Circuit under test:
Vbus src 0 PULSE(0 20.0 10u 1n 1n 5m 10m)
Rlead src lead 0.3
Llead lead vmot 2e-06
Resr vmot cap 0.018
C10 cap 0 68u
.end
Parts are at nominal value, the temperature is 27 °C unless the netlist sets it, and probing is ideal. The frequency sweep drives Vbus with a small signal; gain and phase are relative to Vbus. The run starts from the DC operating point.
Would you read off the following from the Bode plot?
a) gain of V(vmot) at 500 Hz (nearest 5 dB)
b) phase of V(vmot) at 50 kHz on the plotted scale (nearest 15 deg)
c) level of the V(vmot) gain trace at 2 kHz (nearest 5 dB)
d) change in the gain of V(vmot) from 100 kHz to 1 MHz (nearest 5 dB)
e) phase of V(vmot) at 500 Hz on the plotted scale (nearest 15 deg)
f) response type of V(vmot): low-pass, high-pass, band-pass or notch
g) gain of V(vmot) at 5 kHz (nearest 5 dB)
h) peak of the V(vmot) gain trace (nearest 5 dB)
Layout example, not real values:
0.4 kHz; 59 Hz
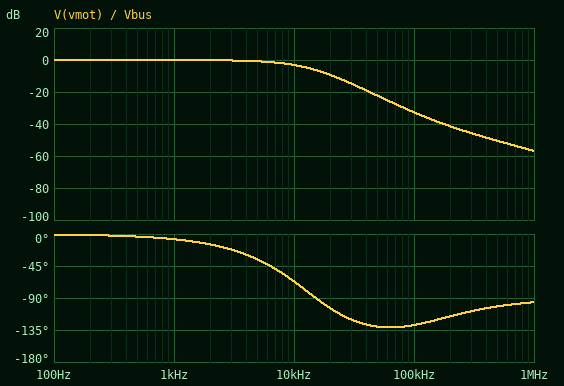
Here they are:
0 dB; -135 deg; 0 dB; -25 dB; 0 deg; low-pass; 0 dB; 0 dB
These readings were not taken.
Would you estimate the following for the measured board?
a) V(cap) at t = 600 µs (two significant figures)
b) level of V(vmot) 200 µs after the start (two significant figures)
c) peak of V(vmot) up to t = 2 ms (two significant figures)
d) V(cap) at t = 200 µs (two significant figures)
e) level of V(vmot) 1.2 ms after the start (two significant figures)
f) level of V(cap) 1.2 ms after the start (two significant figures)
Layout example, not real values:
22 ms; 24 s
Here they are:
20 V; 20 V; 20 V; 20 V; 20 V; 20 V
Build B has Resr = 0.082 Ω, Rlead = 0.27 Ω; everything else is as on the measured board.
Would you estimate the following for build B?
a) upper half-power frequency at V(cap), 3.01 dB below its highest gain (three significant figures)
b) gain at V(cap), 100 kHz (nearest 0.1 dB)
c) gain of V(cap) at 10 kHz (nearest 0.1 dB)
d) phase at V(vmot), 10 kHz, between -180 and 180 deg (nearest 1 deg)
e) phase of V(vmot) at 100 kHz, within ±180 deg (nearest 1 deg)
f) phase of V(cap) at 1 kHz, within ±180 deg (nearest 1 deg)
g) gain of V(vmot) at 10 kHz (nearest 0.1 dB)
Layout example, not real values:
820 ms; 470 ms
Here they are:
8.47 kHz; -34.8 dB; -3.9 dB; -54 deg; -90 deg; -9 deg; -3.4 dB
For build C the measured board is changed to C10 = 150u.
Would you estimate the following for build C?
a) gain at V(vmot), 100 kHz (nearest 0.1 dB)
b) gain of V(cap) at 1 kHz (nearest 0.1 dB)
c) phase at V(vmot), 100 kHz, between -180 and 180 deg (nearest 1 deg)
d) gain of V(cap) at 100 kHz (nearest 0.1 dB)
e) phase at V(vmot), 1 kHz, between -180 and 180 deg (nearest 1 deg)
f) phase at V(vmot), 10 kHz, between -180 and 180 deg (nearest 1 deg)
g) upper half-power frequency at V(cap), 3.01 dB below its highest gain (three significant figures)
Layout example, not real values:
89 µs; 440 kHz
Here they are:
-35.8 dB; -0.3 dB; -106 deg; -41.7 dB; -16 deg; -84 deg; 3.83 kHz
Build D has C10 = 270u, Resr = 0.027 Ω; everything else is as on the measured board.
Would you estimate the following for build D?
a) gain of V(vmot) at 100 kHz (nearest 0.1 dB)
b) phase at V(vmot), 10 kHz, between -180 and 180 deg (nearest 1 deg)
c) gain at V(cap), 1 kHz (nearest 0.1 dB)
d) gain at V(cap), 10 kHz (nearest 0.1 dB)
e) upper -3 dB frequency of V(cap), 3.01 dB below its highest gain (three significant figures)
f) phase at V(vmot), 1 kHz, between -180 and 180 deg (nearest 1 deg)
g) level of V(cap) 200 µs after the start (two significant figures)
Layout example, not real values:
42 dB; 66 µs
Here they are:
-33.4 dB; -77 deg; -1.0 dB; -15.1 dB; 1.94 kHz; -27 deg; 18 V
